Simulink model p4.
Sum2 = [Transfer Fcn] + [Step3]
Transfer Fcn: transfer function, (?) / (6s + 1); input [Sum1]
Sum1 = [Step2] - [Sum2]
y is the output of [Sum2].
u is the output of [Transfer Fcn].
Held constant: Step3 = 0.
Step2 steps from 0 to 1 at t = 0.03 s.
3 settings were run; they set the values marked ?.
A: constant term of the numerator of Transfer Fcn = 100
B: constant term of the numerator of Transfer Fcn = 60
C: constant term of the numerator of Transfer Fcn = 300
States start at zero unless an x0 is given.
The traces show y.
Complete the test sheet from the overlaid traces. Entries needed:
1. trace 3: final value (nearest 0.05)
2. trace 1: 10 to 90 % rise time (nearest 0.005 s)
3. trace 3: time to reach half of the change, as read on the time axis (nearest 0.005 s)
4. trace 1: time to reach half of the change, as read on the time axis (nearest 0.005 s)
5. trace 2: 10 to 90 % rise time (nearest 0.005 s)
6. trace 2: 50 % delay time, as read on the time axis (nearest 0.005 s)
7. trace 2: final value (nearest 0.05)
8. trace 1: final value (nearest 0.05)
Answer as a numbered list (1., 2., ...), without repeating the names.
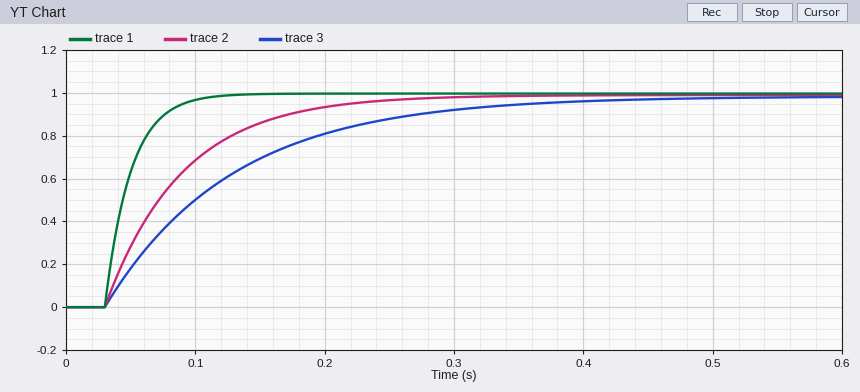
1. 1.00
2. 0.045 s
3. 0.100 s
4. 0.045 s
5. 0.130 s
6. 0.070 s
7. 1.00
8. 1.00
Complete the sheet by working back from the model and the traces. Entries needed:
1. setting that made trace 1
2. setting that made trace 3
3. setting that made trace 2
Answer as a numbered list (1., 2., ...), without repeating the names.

1. C
2. B
3. A
